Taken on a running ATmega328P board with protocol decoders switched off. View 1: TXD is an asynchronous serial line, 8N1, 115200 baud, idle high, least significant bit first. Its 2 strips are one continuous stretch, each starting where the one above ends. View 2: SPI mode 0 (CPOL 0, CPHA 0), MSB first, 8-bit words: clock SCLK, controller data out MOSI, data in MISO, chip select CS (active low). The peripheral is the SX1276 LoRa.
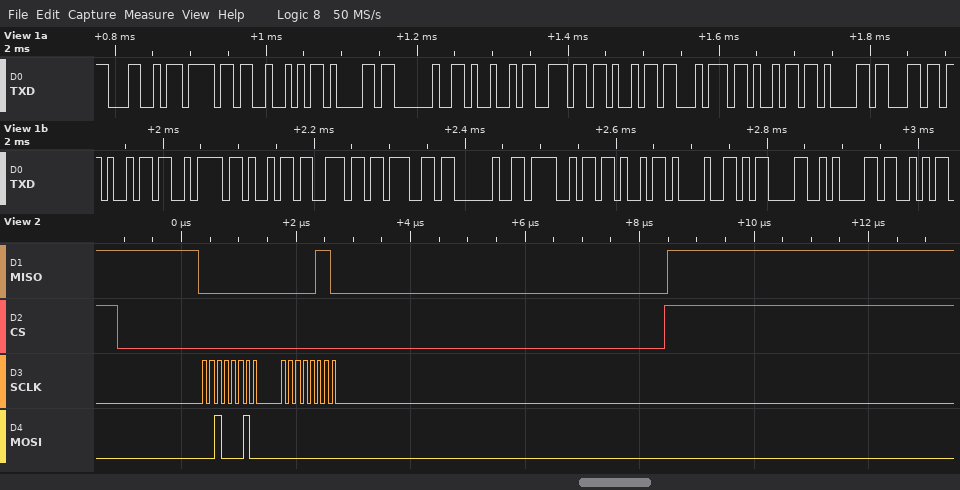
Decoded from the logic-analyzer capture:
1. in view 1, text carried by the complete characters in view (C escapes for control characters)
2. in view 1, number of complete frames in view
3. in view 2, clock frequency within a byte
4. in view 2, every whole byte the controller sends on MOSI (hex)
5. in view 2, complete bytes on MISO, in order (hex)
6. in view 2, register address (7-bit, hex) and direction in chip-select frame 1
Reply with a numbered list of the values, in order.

1. "LoRa Initializing OK!\r\nS"
2. 24
3. 8 MHz
4. 22 00
5. 00 06
6. 0x22 read
